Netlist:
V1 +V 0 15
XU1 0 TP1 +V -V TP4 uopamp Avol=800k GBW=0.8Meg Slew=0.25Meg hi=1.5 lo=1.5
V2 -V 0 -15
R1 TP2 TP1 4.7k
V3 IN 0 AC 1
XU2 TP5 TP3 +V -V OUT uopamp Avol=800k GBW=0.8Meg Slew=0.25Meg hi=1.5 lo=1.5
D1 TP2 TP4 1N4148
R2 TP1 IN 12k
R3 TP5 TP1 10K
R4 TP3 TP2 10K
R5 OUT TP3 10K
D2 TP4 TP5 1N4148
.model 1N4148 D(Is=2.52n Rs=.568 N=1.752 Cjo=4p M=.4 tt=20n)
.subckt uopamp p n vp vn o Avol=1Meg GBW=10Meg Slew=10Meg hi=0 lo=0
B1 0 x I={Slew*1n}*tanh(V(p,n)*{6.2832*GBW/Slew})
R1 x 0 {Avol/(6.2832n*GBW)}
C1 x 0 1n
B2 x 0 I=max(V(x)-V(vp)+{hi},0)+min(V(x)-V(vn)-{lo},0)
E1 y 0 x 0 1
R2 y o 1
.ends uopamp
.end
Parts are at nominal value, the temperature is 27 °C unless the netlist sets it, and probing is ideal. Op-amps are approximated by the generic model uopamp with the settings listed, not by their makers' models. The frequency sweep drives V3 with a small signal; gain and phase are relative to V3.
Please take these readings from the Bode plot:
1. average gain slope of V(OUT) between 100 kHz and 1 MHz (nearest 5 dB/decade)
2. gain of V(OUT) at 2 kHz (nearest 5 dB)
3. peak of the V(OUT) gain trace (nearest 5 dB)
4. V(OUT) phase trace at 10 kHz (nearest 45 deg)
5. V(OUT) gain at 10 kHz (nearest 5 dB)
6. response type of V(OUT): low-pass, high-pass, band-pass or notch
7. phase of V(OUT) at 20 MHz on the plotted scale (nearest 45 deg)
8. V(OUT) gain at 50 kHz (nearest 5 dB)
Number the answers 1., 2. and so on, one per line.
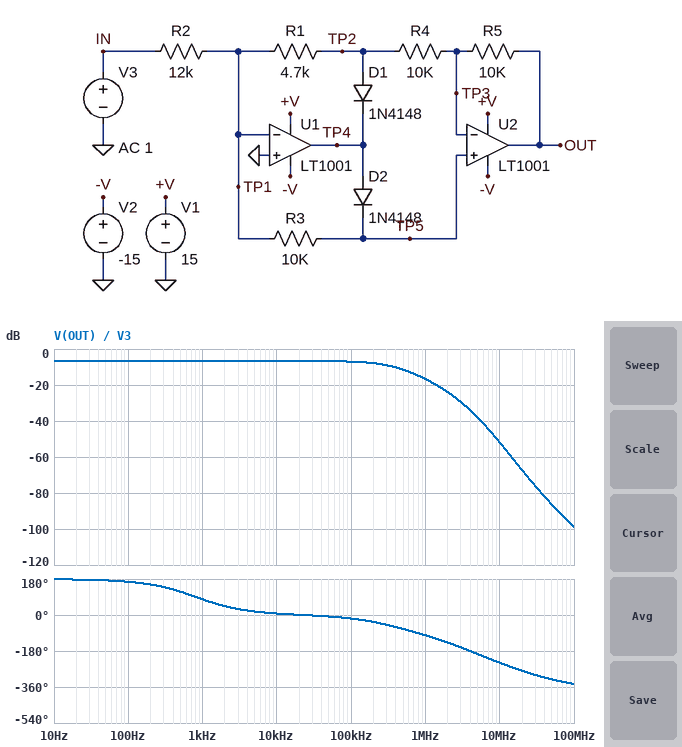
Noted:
1. -10 dB/decade
2. -5 dB
3. -5 dB
4. 0 deg
5. -5 dB
6. low-pass
7. -270 deg
8. -5 dB
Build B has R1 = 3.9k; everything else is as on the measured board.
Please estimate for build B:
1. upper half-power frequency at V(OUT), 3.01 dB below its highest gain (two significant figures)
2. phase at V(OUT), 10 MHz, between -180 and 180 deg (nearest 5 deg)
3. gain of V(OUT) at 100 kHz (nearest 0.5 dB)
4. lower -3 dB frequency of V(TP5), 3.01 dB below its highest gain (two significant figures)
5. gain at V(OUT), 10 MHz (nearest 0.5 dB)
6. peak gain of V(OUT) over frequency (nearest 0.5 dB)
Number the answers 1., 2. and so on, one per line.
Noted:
1. 280 kHz
2. 105 deg
3. -7.5 dB
4. 230 Hz
5. -50.5 dB
6. -6.0 dB
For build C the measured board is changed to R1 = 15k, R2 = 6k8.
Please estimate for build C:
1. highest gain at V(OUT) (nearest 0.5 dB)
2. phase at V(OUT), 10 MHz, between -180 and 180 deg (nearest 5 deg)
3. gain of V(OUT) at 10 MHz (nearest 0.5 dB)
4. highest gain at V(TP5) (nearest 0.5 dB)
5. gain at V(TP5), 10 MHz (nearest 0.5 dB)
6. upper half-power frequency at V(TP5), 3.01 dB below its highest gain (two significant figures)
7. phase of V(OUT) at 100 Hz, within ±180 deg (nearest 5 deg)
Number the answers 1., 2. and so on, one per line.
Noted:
1. -3.5 dB
2. -165 deg
3. -41.5 dB
4. -2.0 dB
5. -17.0 dB
6. 550 kHz
7. 155 deg
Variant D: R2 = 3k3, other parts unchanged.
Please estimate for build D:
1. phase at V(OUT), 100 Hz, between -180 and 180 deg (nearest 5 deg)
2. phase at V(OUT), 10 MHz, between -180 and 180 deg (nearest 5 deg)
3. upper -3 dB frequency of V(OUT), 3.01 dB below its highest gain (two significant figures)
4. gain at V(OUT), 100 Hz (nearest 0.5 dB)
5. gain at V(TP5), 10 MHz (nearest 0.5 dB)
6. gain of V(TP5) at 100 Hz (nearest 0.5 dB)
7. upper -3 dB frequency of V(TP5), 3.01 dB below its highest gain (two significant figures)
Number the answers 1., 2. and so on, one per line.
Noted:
1. 155 deg
2. 130 deg
3. 350 Hz
4. 4.5 dB
5. -15.5 dB
6. 2.0 dB
7. 470 Hz
